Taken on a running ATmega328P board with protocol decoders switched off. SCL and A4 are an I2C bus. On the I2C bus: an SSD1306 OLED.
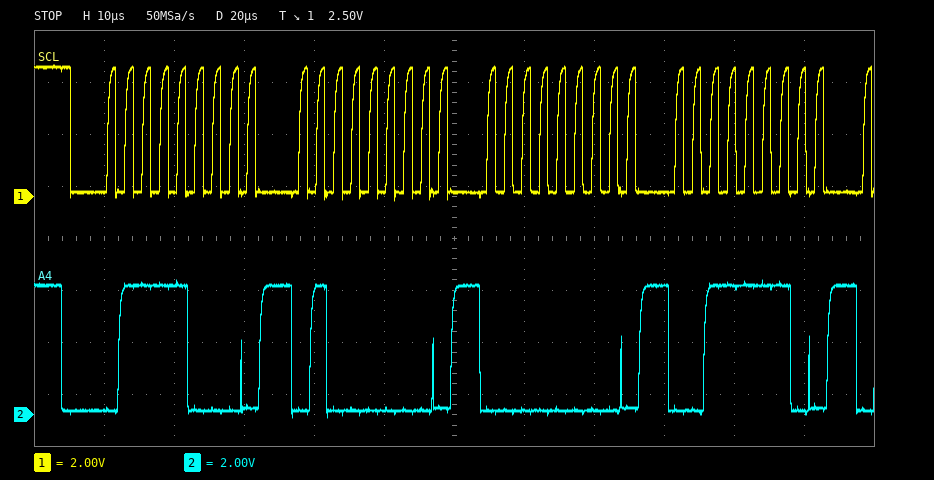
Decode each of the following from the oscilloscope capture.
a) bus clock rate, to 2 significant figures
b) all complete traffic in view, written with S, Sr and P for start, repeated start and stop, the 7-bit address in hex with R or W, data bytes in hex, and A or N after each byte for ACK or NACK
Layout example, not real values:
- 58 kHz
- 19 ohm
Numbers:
- 400 kHz
- S 3CW A 40 A 00 A 3E A
